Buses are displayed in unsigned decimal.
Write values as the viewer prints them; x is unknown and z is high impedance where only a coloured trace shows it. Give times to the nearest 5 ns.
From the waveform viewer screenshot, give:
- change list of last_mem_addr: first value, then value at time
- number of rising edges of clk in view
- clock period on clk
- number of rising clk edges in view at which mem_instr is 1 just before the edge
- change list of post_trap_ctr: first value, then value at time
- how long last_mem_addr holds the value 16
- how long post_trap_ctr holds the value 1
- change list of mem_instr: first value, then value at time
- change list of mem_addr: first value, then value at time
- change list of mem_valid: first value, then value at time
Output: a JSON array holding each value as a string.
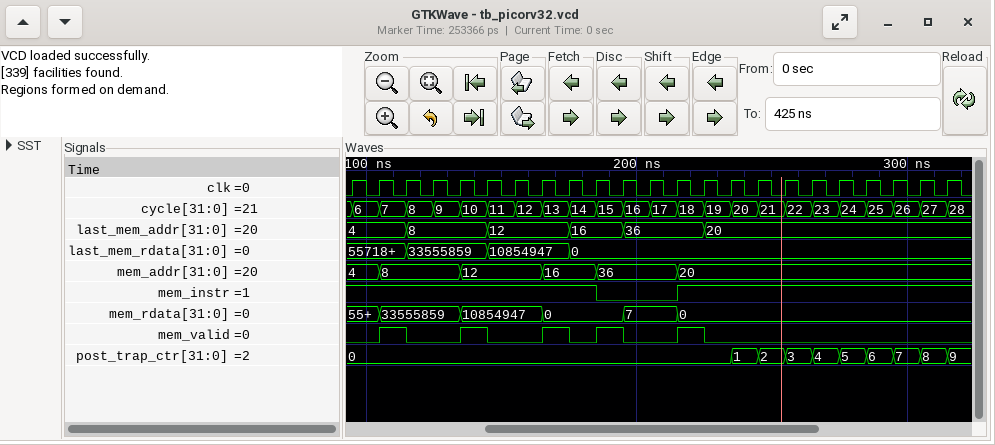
["4, 8 at 115 ns, 12 at 145 ns, 16 at 175 ns, 36 at 195 ns, 20 at 225 ns", "23", "10 ns", "20", "0, 1 at 235 ns, 2 at 245 ns, 3 at 255 ns, 4 at 265 ns, 5 at 275 ns, 6 at 285 ns, 7 at 295 ns, 8 at 305 ns, 9 at 315 ns", "20 ns", "10 ns", "1, 0 at 185 ns, 1 at 215 ns", "4, 8 at 105 ns, 12 at 135 ns, 16 at 165 ns, 36 at 185 ns, 20 at 215 ns", "0, 1 at 105 ns, 0 at 115 ns, 1 at 135 ns, 0 at 145 ns, 1 at 165 ns, 0 at 175 ns, 1 at 185 ns, 0 at 195 ns, 1 at 215 ns, 0 at 225 ns"]
